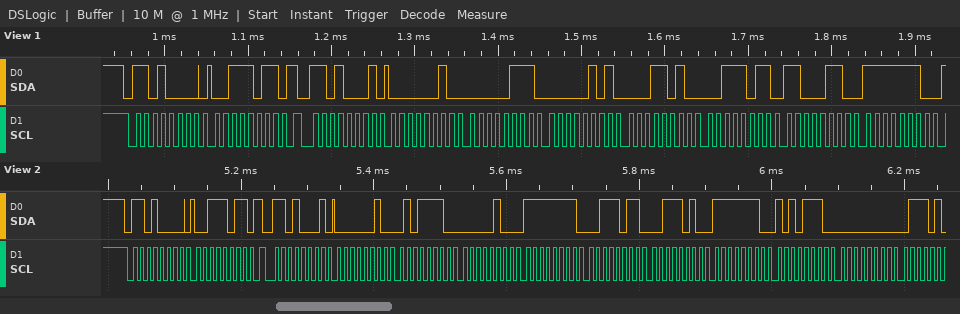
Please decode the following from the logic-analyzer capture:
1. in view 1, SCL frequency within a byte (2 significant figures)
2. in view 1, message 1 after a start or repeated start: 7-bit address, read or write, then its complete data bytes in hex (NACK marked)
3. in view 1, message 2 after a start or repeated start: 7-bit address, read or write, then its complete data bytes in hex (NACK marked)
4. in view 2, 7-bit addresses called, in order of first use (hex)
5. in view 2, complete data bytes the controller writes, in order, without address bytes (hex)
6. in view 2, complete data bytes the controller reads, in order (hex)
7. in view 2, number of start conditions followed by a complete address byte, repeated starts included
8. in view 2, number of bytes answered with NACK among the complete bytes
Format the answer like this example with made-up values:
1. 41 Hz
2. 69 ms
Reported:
1. 100 kHz
2. 0x68 write: 3B
3. 0x68 read: 02 07 05 1A 3B C6 FE
4. 0x68
5. 3B
6. 02 5E 04 FF 3B 3A FE AE 00
7. 2
8. 0
